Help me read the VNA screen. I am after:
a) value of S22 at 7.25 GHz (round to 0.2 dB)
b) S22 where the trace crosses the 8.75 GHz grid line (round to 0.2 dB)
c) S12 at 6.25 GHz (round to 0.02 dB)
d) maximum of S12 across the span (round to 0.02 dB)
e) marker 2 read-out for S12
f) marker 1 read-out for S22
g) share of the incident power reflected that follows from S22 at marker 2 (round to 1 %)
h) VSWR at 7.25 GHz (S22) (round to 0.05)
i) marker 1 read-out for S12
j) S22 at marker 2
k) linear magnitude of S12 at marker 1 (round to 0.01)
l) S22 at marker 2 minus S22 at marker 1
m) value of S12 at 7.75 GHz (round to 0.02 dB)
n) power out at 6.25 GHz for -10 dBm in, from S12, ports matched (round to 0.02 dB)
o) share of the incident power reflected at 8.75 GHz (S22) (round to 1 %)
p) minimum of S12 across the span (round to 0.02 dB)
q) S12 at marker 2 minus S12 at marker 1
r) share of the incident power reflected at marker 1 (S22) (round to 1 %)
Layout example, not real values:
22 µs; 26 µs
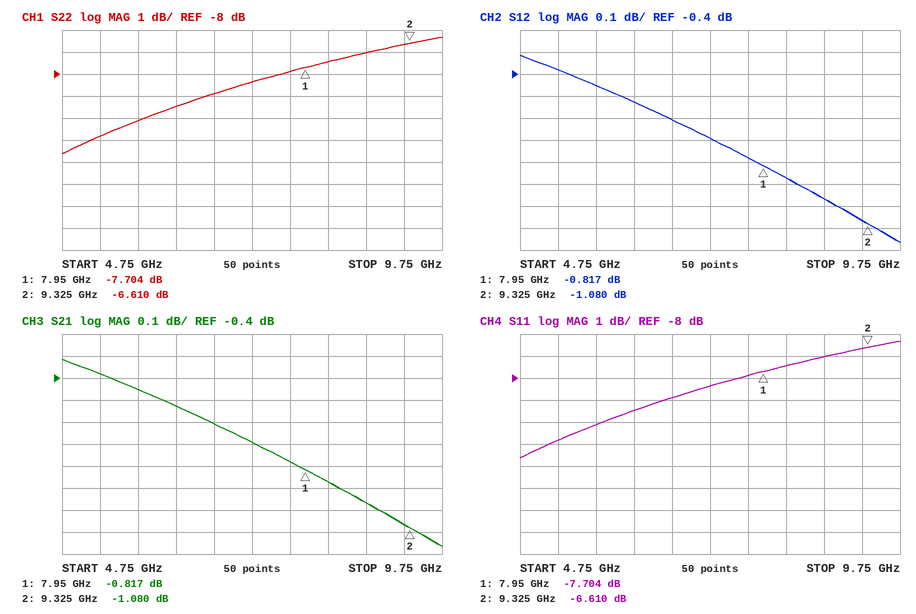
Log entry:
-8.4 dB; -7.0 dB; -0.52 dB; -0.32 dB; -1.080 dB; -7.704 dB; 22 %; 2.25; -0.817 dB; -6.610 dB; 0.91; 1.094 dB; -0.78 dB; -10.52 dBm; 20 %; -1.16 dB; -0.263 dB; 17 %
